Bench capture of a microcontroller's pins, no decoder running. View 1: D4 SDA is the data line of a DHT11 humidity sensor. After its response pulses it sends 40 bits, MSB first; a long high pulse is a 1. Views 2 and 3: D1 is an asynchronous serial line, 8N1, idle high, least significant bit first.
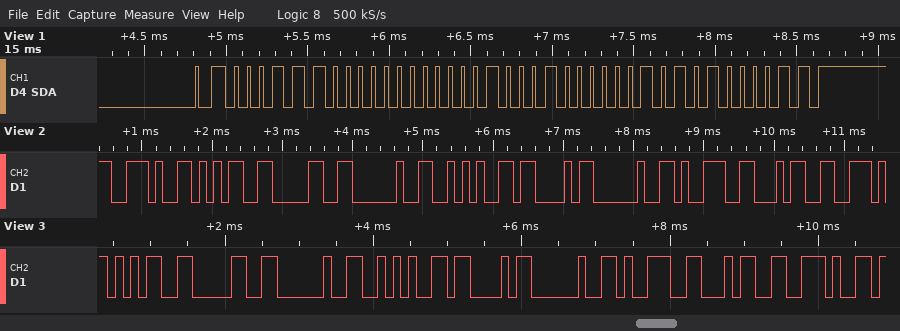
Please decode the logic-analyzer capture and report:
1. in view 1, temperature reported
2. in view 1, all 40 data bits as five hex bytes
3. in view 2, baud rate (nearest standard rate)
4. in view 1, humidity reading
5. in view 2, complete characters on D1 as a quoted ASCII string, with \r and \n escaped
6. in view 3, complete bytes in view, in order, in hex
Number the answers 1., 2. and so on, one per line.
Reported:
1. 34.5 °C
2. 1C 00 22 05 43
3. 9600 baud
4. 28 %
5. ".50 *C 94"
6. 35 30 20 2A 43 20 39 34 2E
